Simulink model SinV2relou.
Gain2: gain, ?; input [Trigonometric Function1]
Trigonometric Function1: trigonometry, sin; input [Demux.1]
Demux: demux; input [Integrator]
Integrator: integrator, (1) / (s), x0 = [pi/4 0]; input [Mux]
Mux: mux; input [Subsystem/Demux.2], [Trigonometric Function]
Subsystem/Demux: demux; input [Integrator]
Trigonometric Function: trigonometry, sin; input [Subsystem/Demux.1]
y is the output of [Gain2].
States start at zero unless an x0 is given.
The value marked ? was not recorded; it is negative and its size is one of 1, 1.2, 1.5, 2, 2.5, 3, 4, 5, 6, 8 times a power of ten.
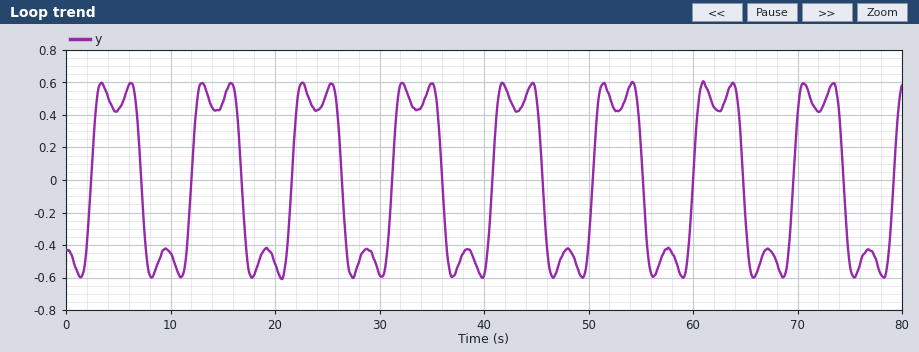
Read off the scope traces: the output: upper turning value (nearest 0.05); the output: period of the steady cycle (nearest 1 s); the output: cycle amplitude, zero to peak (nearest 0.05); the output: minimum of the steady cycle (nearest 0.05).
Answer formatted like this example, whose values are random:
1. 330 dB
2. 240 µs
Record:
1. 0.60
2. 10 s
3. 0.60
4. -0.60
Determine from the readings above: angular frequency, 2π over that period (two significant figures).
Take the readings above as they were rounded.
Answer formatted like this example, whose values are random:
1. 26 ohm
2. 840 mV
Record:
1. 0.63 rad/s
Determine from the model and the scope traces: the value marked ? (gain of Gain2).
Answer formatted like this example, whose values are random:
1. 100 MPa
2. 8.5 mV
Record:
1. -0.6
